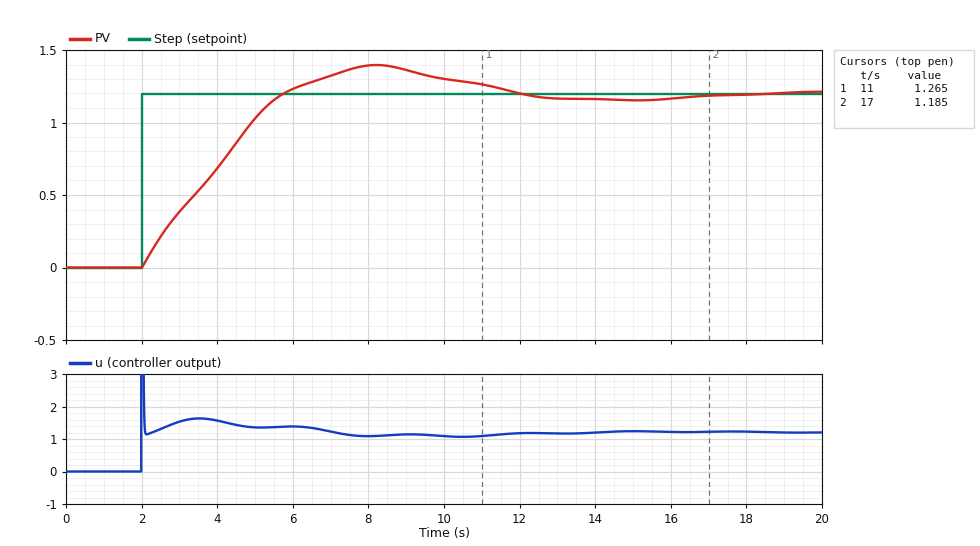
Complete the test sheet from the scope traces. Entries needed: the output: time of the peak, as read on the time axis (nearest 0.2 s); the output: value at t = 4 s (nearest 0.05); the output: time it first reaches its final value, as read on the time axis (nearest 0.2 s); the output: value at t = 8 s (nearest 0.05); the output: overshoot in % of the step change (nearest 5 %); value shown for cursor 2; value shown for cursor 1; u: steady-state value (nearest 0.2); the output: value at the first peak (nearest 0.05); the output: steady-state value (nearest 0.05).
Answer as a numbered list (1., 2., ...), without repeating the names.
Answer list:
1. 8.2 s
2. 0.70
3. 5.8 s
4. 1.40
5. 15 %
6. 1.185
7. 1.265
8. 1.2
9. 1.40
10. 1.20
